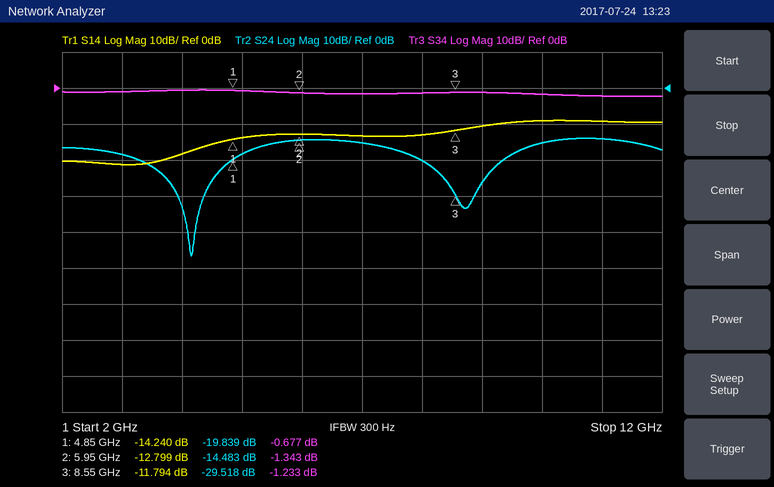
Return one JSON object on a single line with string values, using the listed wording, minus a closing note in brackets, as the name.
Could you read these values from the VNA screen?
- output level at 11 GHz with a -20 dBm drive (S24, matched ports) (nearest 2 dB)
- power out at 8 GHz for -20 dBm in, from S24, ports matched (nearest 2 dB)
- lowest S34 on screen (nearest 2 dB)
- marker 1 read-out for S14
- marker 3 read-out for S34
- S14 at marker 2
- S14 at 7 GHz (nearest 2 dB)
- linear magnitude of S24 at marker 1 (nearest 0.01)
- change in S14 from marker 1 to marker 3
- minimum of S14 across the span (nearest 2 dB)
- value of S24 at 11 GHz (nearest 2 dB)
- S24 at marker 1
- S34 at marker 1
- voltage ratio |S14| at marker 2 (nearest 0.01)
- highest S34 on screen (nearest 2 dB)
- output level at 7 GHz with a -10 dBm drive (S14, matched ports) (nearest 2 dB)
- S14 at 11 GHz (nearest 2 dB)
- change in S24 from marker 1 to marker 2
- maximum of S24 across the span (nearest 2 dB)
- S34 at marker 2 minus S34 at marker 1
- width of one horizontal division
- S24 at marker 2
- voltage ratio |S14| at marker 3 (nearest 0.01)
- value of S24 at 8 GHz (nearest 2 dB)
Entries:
{"output level at 11 GHz with a -20 dBm drive (S24, matched ports)": "-34 dBm", "power out at 8 GHz for -20 dBm in, from S24, ports matched": "-40 dBm", "lowest S34 on screen": "-2 dB", "marker 1 read-out for S14": "-14.240 dB", "marker 3 read-out for S34": "-1.233 dB", "S14 at marker 2": "-12.799 dB", "S14 at 7 GHz": "-14 dB", "linear magnitude of S24 at marker 1": "0.10", "change in S14 from marker 1 to marker 3": "2.446 dB", "minimum of S14 across the span": "-22 dB", "value of S24 at 11 GHz": "-14 dB", "S24 at marker 1": "-19.839 dB", "S34 at marker 1": "-0.677 dB", "voltage ratio |S14| at marker 2": "0.23", "highest S34 on screen": "0 dB", "output level at 7 GHz with a -10 dBm drive (S14, matched ports)": "-24 dBm", "S14 at 11 GHz": "-10 dB", "change in S24 from marker 1 to marker 2": "5.356 dB", "maximum of S24 across the span": "-14 dB", "S34 at marker 2 minus S34 at marker 1": "-0.666 dB", "width of one horizontal division": "1 GHz", "S24 at marker 2": "-14.483 dB", "voltage ratio |S14| at marker 3": "0.26", "value of S24 at 8 GHz": "-20 dB"}
